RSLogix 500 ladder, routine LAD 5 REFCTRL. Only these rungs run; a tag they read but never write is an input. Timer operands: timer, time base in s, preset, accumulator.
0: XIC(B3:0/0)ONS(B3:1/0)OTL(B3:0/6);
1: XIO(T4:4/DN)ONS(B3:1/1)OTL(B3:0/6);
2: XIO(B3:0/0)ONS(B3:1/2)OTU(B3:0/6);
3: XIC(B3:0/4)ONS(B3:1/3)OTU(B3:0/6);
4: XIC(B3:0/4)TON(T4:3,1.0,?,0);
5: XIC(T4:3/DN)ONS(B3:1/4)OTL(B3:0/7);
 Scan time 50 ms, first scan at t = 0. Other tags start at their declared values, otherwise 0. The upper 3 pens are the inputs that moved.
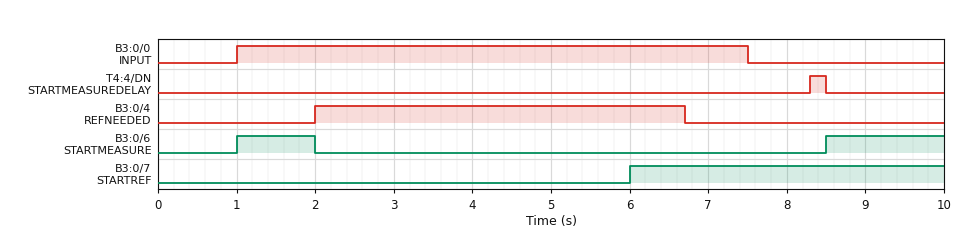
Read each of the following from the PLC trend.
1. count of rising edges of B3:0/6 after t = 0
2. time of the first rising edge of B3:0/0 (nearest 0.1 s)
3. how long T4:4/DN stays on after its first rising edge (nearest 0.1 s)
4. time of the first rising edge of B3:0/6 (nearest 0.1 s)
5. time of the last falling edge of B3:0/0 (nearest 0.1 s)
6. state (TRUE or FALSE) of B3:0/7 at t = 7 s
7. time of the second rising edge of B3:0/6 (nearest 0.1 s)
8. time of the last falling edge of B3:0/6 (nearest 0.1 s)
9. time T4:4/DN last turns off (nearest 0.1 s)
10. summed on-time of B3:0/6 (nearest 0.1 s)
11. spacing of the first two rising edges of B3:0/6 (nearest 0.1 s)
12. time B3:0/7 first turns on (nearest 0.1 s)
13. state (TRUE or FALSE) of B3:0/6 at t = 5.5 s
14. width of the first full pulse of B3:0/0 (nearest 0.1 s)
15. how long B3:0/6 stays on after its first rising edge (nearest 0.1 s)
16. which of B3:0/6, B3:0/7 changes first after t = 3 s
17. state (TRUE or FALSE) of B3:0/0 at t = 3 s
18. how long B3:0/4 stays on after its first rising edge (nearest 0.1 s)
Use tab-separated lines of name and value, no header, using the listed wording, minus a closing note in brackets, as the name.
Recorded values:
count of rising edges of B3:0/6 after t = 0	2
time of the first rising edge of B3:0/0	1.0 s
how long T4:4/DN stays on after its first rising edge	0.2 s
time of the first rising edge of B3:0/6	1.0 s
time of the last falling edge of B3:0/0	7.5 s
state (TRUE or FALSE) of B3:0/7 at t = 7 s	TRUE
time of the second rising edge of B3:0/6	8.5 s
time of the last falling edge of B3:0/6	2.0 s
time T4:4/DN last turns off	8.5 s
summed on-time of B3:0/6	2.5 s
spacing of the first two rising edges of B3:0/6	7.5 s
time B3:0/7 first turns on	6.0 s
state (TRUE or FALSE) of B3:0/6 at t = 5.5 s	FALSE
width of the first full pulse of B3:0/0	6.5 s
how long B3:0/6 stays on after its first rising edge	1.0 s
which of B3:0/6, B3:0/7 changes first after t = 3 s	B3:0/7
state (TRUE or FALSE) of B3:0/0 at t = 3 s	TRUE
how long B3:0/4 stays on after its first rising edge	4.7 s
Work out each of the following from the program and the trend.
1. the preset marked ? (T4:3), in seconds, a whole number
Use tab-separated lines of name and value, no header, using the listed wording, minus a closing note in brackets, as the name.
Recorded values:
the preset marked ? (T4:3), in seconds, a whole number	4 s
